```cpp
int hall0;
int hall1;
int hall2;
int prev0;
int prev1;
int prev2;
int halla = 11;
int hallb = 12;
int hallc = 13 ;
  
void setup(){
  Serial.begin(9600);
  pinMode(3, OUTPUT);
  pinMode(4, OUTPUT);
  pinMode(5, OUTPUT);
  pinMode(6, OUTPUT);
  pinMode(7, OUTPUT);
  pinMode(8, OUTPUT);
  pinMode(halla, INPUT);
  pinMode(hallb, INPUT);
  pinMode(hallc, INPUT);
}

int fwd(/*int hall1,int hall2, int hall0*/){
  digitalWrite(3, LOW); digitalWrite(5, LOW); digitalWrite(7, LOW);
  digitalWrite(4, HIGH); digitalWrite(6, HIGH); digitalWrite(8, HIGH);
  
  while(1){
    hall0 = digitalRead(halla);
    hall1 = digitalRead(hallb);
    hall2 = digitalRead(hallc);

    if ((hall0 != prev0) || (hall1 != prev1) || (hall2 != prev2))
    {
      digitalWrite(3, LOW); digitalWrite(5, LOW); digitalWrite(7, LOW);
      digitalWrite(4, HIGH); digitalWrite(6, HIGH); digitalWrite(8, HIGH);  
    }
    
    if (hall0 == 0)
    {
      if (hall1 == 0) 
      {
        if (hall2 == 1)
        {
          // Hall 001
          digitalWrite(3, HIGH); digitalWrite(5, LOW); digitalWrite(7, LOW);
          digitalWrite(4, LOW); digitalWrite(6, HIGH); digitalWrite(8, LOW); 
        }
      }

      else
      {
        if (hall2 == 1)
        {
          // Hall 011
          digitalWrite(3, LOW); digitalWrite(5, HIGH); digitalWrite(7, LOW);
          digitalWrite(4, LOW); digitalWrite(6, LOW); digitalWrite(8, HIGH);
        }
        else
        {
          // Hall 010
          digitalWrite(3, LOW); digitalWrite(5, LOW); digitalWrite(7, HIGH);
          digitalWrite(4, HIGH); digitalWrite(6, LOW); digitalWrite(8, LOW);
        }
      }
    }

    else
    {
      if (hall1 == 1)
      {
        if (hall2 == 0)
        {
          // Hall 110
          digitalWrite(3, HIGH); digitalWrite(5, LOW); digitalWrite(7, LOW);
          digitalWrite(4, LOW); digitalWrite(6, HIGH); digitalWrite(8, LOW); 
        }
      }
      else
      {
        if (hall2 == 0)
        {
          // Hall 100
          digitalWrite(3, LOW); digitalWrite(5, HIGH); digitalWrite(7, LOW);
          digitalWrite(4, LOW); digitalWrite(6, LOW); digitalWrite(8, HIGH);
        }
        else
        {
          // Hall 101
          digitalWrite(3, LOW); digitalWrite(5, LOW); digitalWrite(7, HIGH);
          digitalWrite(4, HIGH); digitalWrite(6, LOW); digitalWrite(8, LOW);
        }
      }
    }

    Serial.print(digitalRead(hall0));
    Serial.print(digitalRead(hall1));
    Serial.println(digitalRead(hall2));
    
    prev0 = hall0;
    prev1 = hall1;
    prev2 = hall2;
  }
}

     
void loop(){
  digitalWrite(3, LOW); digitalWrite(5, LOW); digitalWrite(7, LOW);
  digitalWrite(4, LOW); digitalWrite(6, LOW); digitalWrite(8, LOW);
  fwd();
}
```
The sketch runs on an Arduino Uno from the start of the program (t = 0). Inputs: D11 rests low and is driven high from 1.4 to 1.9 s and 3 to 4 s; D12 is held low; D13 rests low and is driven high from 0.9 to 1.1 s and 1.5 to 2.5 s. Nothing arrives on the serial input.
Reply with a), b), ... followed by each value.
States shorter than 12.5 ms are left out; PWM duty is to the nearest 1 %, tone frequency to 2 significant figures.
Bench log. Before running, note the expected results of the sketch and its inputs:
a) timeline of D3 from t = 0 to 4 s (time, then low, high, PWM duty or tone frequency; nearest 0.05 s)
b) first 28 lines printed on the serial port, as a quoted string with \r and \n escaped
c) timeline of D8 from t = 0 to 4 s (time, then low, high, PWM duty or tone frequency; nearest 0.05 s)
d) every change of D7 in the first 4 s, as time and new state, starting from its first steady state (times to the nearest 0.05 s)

a) 0 s low; 0.9 s high; 1.1 s low; 1.9 s high; 2.5 s low
b) "000\r\n000\r\n000\r\n000\r\n000\r\n000\r\n000\r\n000\r\n000\r\n000\r\n000\r\n000\r\n000\r\n000\r\n000\r\n000\r\n000\r\n000\r\n000\r\n000\r\n000\r\n000\r\n000\r\n000\r\n000\r\n000\r\n000\r\n000\r\n"
c) 0 s high; 0.9 s low; 1.1 s high; 1.5 s low; 2.5 s high
d) 0 s low; 1.5 s high; 1.9 s low
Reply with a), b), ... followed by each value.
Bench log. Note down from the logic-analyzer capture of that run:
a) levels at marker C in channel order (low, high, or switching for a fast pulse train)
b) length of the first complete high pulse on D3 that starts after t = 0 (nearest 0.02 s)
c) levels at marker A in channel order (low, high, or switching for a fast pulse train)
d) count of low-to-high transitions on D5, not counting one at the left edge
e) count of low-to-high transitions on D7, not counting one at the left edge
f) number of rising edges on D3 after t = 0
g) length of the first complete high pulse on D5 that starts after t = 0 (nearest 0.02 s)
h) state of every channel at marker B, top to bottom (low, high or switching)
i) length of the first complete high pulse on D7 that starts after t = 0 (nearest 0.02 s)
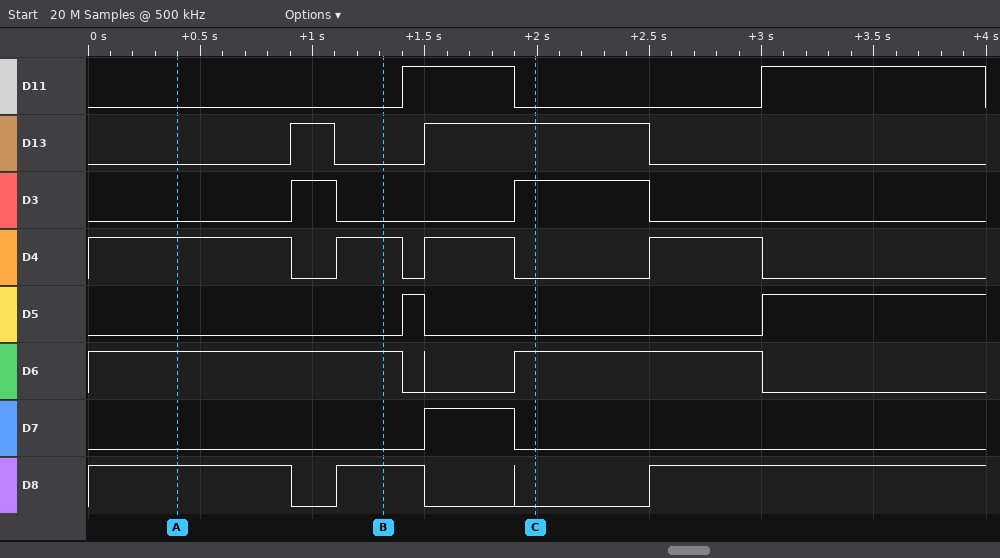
a) D11 low, D13 high, D3 high, D4 low, D5 low, D6 high, D7 low, D8 low
b) 0.20 s
c) D11 low, D13 low, D3 low, D4 high, D5 low, D6 high, D7 low, D8 high
d) 2
e) 1
f) 2
g) 0.10 s
h) D11 low, D13 low, D3 low, D4 high, D5 low, D6 high, D7 low, D8 high
i) 0.40 s
